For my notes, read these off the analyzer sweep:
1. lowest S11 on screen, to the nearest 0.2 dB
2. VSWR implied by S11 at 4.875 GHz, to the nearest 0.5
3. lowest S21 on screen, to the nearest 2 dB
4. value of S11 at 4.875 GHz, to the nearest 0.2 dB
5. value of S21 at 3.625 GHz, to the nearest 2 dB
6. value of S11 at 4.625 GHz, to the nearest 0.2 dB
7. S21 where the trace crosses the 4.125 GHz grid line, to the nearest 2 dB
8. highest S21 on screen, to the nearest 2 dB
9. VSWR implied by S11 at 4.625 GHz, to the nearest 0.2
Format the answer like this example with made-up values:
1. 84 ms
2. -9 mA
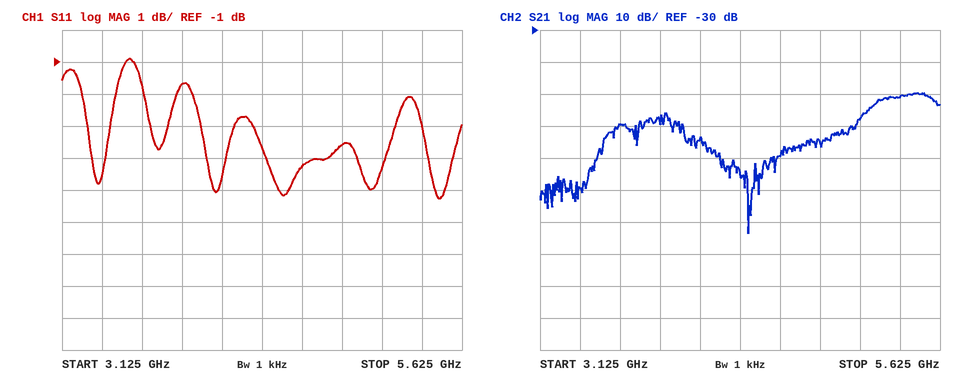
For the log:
1. -5.2 dB
2. 5.0
3. -94 dB
4. -3.6 dB
5. -60 dB
6. -4.2 dB
7. -64 dB
8. -50 dB
9. 4.2
